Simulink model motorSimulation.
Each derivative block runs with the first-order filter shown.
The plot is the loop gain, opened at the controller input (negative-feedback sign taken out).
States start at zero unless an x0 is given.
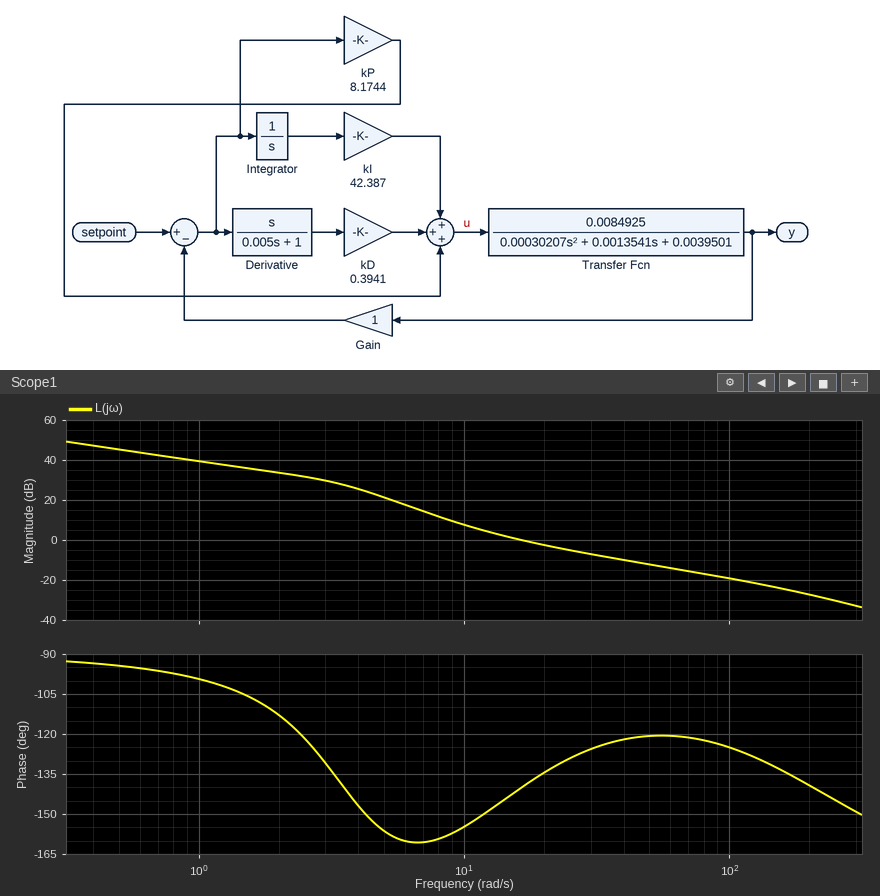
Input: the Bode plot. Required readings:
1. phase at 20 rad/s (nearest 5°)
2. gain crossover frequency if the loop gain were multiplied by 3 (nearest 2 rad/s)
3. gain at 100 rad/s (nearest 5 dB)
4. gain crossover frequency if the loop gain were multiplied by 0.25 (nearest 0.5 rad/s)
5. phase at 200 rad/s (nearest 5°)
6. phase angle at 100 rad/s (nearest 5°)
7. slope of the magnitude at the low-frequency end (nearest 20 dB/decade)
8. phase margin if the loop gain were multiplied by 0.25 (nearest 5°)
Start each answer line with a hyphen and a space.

- -135°
- 38 rad/s
- -20 dB
- 8.0 rad/s
- -140°
- -125°
- -20 dB/decade
- 20°
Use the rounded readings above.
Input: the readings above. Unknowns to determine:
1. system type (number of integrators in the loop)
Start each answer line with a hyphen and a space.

- 1
